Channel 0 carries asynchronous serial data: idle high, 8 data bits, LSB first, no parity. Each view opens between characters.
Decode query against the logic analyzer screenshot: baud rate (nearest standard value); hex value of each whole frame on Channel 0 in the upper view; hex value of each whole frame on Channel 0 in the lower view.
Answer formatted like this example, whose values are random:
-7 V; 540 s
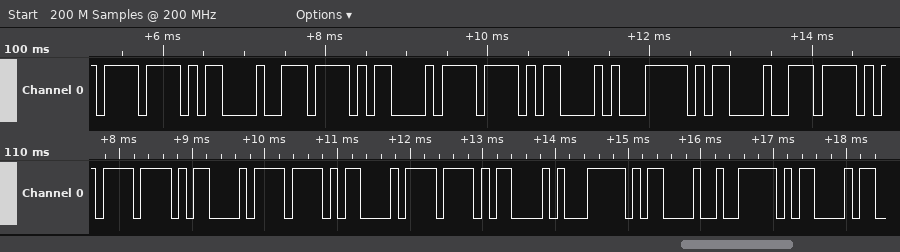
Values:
9600 baud; EF, 0D, EE, 0D, EF, 0D, F1, 0D, EE; EF, 0D, EF, 0D, EF, 0D, F1, 0D, F2, 0D
